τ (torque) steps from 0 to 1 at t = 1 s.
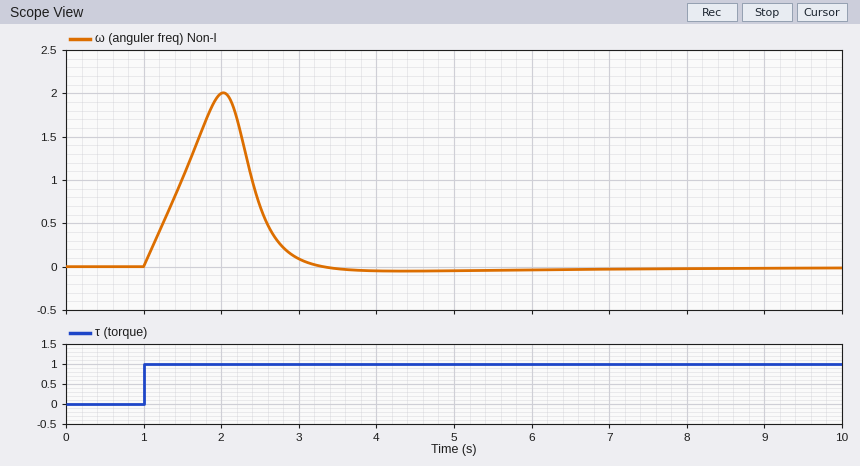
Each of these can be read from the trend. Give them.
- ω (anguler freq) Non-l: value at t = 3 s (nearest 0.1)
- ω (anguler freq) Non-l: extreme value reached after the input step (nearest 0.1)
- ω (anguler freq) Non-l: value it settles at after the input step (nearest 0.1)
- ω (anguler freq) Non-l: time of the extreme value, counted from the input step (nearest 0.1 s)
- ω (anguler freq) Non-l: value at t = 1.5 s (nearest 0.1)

0.1
2.0
0.0
1.0 s
1.0
